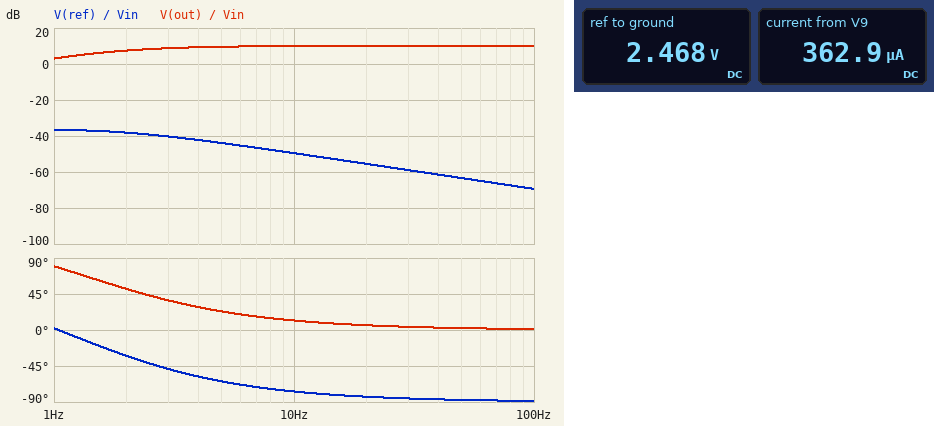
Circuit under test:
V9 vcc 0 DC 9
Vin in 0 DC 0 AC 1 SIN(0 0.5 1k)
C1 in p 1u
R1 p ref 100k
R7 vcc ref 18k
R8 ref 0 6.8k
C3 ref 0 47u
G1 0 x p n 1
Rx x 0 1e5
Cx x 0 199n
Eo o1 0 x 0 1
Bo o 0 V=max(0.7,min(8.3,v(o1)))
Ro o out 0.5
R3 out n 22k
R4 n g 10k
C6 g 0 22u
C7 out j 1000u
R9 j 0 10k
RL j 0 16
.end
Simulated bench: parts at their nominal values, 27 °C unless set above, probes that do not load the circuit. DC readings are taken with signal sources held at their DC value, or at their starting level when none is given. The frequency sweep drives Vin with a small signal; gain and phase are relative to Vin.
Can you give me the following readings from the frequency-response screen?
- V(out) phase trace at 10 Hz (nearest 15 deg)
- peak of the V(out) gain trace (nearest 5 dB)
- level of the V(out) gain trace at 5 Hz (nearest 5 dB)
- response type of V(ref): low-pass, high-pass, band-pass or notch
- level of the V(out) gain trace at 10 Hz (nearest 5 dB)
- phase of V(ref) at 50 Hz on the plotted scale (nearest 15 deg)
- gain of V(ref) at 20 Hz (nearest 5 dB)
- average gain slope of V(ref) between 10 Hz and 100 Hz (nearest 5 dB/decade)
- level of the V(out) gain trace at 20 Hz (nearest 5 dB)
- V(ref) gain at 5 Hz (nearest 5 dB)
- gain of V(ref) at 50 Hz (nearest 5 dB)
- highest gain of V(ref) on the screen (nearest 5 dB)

15 deg
10 dB
10 dB
low-pass
10 dB
-90 deg
-55 dB
-20 dB/decade
10 dB
-45 dB
-65 dB
-35 dB
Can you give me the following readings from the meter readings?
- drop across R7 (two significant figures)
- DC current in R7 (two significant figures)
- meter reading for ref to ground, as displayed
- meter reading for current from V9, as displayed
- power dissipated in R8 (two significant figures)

6.5 V
360 µA
2.468 V
362.9 µA
900 µW
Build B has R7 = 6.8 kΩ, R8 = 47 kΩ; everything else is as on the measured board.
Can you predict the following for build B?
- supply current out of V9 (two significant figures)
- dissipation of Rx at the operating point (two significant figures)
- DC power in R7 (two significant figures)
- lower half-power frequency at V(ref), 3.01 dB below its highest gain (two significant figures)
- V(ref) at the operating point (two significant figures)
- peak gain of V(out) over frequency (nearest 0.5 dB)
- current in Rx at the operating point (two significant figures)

170 µA
620 µW
190 µW
360 mHz
7.9 V
10.0 dB
79 µA
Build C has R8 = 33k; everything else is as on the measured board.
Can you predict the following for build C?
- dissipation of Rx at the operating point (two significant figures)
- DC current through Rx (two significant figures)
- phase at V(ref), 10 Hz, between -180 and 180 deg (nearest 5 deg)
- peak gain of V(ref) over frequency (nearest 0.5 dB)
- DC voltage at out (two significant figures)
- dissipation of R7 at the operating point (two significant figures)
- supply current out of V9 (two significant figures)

340 µW
58 µA
-80 deg
-35.0 dB
5.8 V
560 µW
180 µA
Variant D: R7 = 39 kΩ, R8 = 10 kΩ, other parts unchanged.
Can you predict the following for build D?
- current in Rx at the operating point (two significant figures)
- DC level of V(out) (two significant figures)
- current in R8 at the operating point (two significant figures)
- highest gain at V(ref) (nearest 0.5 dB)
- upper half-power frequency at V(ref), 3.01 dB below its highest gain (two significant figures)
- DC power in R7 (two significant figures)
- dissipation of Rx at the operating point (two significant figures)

18 µA
1.8 V
180 µA
-35.5 dB
2.3 Hz
1.3 mW
34 µW
